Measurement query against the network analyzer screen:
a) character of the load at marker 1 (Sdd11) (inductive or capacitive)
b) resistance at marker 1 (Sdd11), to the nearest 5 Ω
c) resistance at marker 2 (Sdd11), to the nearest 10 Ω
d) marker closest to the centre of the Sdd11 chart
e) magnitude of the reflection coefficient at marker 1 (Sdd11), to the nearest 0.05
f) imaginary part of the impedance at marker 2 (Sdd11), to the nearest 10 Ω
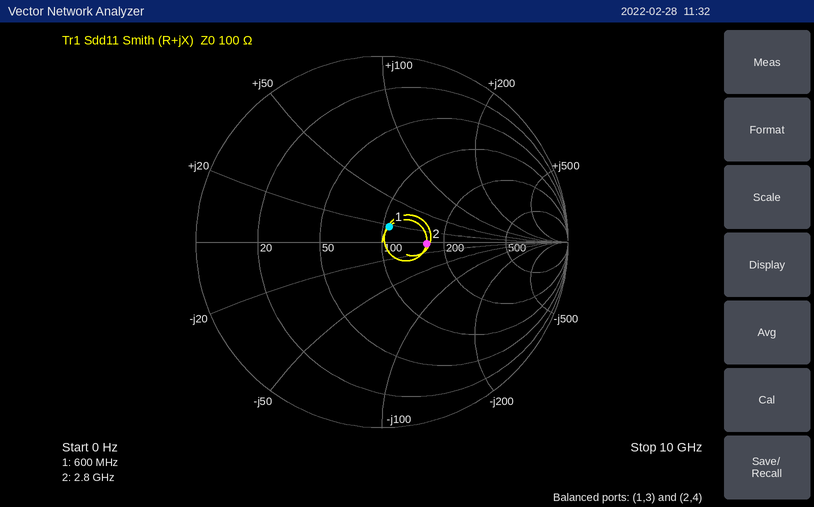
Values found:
inductive
105 Ω
160 Ω
marker 1
0.10
0 Ω
